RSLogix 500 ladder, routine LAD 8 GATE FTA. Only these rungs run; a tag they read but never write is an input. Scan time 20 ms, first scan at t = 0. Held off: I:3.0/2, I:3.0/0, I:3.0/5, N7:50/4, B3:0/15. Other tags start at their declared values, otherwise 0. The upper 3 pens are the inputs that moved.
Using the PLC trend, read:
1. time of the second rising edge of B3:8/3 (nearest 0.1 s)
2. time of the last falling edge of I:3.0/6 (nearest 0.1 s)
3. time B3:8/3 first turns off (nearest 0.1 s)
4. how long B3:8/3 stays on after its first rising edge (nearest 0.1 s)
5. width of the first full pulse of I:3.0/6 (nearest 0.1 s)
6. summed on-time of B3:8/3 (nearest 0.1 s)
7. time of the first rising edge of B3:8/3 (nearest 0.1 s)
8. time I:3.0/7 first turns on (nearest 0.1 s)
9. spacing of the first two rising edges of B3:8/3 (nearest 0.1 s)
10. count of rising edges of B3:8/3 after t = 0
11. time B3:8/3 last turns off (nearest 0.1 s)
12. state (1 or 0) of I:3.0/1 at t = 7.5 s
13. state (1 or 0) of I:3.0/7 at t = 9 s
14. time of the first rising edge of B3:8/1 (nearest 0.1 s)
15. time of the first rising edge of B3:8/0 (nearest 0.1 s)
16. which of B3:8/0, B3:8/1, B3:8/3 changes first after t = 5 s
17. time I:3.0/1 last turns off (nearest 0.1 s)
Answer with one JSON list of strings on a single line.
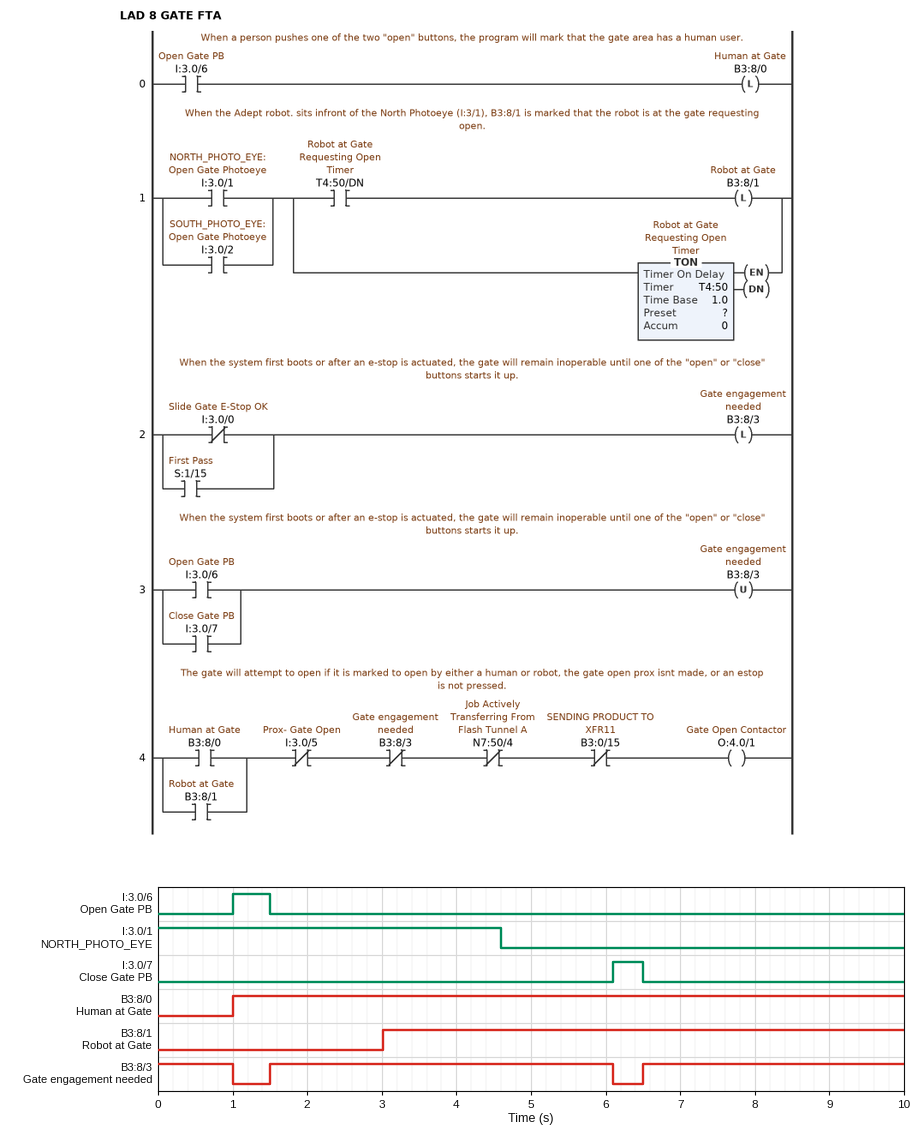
["6.5 s", "1.5 s", "1.0 s", "4.6 s", "0.5 s", "9.1 s", "1.5 s", "6.1 s", "5.0 s", "2", "6.1 s", "0", "0", "3.0 s", "1.0 s", "B3:8/3", "4.6 s"]
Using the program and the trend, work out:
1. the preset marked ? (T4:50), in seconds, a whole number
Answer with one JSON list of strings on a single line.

["3 s"]
